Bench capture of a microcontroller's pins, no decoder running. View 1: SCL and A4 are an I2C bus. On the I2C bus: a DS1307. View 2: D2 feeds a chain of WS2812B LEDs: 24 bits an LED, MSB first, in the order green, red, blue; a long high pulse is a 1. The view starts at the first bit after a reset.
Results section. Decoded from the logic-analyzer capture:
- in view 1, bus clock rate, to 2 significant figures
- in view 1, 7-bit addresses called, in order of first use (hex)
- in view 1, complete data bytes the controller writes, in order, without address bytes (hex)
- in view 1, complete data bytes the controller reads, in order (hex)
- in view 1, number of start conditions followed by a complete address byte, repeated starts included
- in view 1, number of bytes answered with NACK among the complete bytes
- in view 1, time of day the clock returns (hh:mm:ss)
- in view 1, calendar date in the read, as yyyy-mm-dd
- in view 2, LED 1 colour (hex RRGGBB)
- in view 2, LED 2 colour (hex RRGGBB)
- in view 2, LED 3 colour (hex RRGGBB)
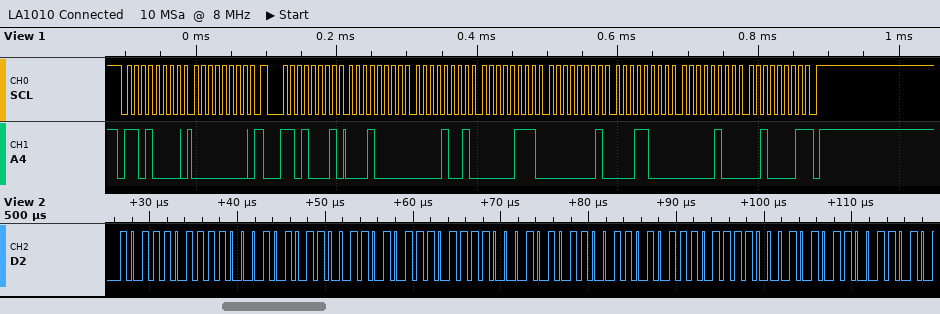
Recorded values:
100 kHz
0x68
00
10 09 07 01 18 04 21
2
1
07:09:10
2021-04-18
#C5BB66
#C5BB66
#C5BB66
